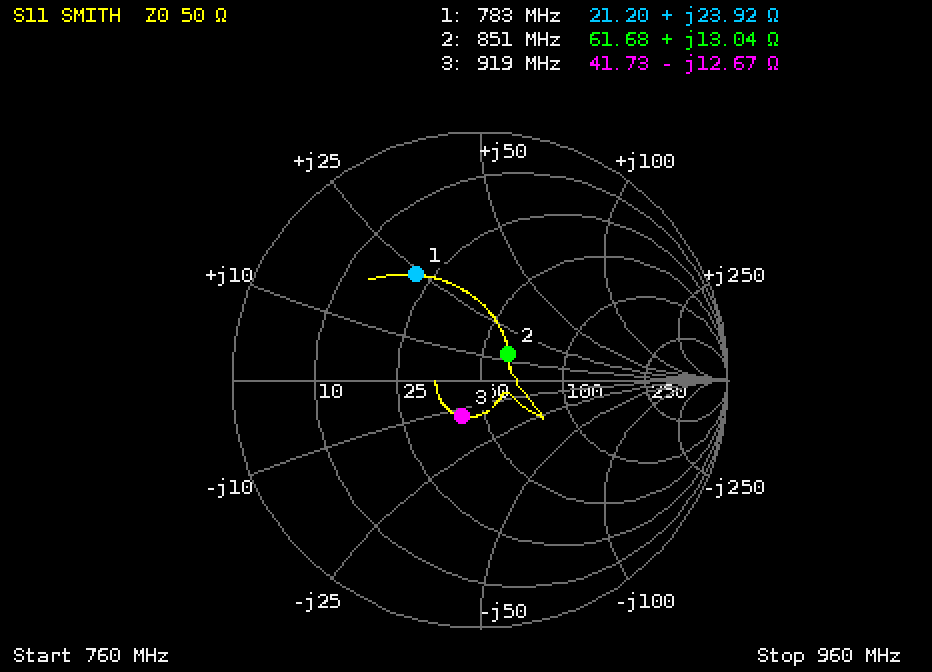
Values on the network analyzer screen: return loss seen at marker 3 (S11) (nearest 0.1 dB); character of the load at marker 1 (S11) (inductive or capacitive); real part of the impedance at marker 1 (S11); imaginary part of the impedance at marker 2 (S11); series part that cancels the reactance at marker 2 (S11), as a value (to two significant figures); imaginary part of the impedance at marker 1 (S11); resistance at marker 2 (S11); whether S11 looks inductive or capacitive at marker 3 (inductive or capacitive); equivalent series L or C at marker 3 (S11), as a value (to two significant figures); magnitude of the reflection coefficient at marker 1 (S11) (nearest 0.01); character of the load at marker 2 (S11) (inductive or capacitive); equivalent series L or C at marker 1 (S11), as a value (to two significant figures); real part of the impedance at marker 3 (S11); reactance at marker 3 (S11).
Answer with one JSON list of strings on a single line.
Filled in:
["15.7 dB", "inductive", "21.20 Ω", "+13.04 Ω", "14 pF", "+23.92 Ω", "61.68 Ω", "capacitive", "14 pF", "0.50", "inductive", "4.9 nH", "41.73 Ω", "-12.67 Ω"]
